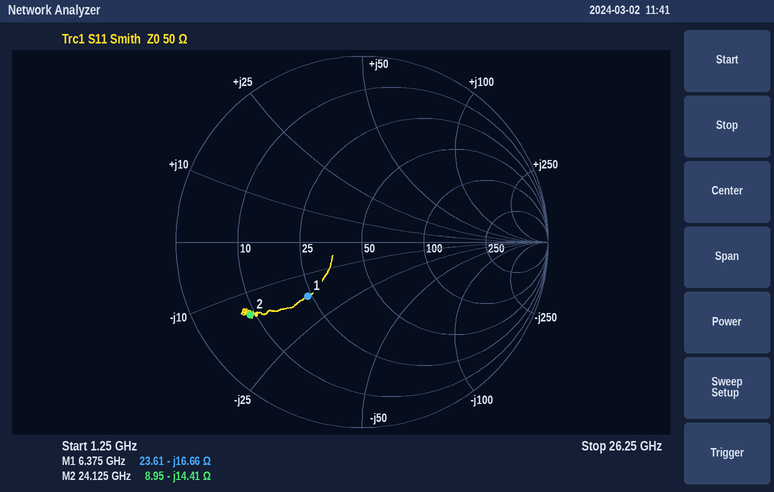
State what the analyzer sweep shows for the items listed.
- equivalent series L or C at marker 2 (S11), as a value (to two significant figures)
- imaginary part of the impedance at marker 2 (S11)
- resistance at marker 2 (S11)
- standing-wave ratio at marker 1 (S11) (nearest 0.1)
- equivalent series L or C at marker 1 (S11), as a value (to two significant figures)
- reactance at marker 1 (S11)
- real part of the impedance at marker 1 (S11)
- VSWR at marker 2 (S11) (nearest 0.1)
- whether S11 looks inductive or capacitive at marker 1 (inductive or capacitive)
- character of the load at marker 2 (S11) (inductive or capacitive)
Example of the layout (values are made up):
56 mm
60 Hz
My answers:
460 fF
-14.41 Ω
8.95 Ω
2.4
1.5 pF
-16.66 Ω
23.61 Ω
6.1
capacitive
capacitive
